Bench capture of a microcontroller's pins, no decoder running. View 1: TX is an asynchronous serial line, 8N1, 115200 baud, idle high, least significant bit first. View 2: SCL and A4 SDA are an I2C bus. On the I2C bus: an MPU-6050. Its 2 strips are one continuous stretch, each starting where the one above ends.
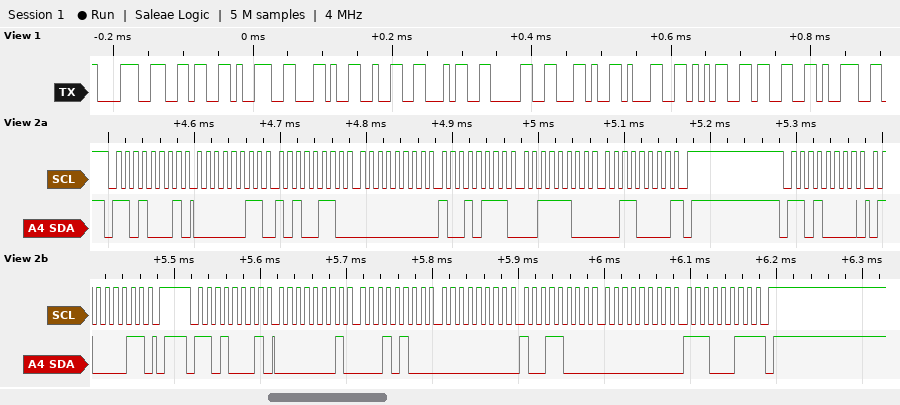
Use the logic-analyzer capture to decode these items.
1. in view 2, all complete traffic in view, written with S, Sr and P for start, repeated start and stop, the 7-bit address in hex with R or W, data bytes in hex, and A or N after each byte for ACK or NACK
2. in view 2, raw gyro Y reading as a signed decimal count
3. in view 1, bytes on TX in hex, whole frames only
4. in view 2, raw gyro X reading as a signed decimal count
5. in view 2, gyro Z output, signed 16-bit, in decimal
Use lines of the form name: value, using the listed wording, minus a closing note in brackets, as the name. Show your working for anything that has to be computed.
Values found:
in view 2, all complete traffic in view, written with S, Sr and P for start, repeated start and stop, the 7-bit address in hex with R or W, data bytes in hex, and A or N after each byte for ACK or NACK: S 68R A 03 A A6 A 00 A 97 A 3C A 30 N P S 68W A 43 A P S 68R A 01 A 14 A 00 A 98 A 00 A E3 N P
in view 2, raw gyro Y reading as a signed decimal count: 0x0098 = 152
in view 1, bytes on TX in hex, whole frames only: 38 36 39 2C 32 34 30 2C 31 35 33 39
in view 2, raw gyro X reading as a signed decimal count: 0x0114 = 276
in view 2, gyro Z output, signed 16-bit, in decimal: 0x00E3 = 227
